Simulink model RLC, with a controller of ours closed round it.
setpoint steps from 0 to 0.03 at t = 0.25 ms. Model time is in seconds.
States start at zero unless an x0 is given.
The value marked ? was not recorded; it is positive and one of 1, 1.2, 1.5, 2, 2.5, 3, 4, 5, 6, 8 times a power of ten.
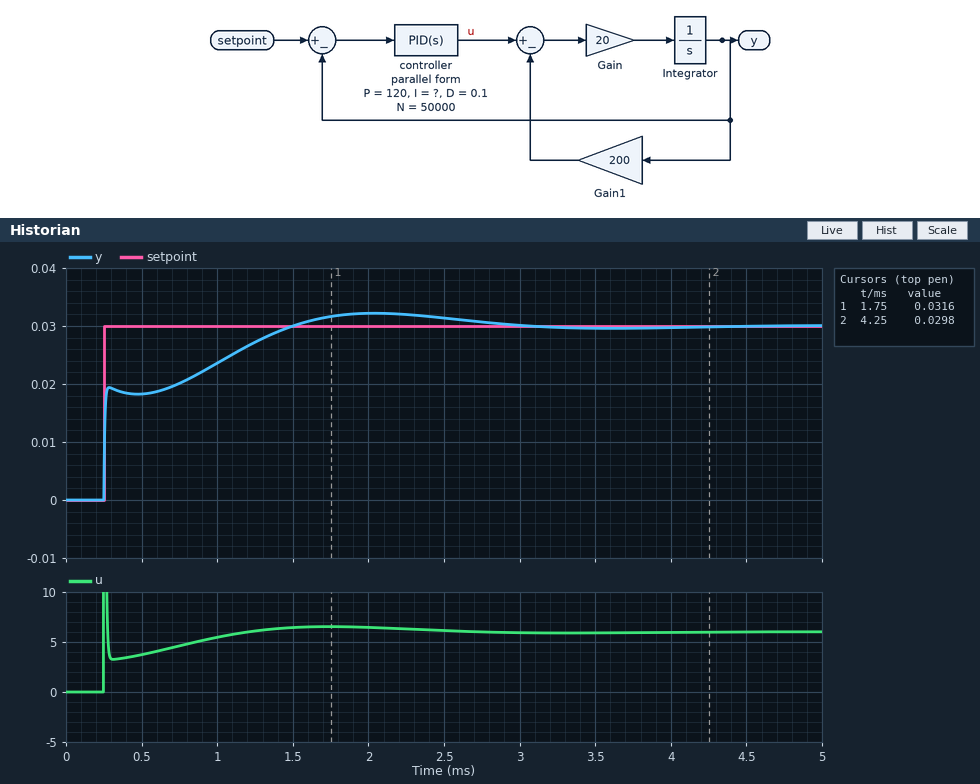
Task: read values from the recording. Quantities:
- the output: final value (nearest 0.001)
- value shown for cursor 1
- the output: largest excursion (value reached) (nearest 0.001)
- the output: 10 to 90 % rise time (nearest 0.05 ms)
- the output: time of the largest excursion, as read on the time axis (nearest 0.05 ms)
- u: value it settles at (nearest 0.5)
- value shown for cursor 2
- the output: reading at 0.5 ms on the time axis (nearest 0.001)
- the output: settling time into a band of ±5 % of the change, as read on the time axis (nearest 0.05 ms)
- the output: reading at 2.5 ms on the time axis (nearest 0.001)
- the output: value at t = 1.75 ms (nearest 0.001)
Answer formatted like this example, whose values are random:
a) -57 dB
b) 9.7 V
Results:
a) 0.030
b) 0.0316
c) 0.032
d) 1.00 ms
e) 2.05 ms
f) 6.0
g) 0.0298
h) 0.018
i) 2.45 ms
j) 0.031
k) 0.032
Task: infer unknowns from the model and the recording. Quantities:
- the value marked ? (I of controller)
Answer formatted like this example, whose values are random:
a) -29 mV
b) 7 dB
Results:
a) 800000
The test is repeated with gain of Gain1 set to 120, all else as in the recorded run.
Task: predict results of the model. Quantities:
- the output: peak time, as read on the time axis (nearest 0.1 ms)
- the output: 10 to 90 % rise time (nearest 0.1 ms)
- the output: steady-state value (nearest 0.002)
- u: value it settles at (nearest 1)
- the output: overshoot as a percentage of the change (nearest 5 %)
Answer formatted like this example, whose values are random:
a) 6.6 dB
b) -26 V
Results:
a) 1.8 ms
b) 0.8 ms
c) 0.030
d) 4
e) 10 %
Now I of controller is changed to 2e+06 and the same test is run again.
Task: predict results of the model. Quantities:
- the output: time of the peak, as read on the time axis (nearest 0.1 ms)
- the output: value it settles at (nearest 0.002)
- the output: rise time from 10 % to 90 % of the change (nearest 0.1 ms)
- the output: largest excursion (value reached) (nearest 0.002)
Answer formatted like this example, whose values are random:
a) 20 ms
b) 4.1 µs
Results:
a) 1.3 ms
b) 0.030
c) 0.5 ms
d) 0.034
